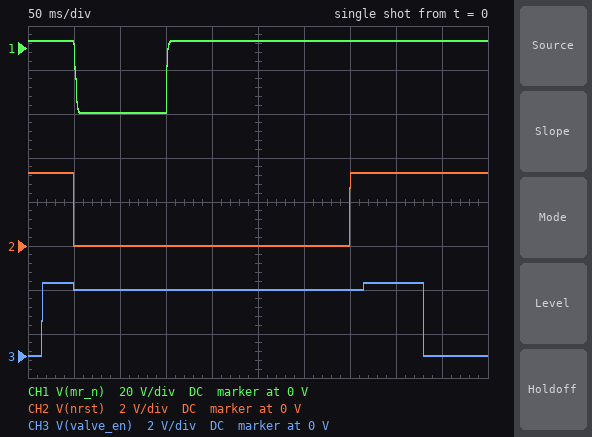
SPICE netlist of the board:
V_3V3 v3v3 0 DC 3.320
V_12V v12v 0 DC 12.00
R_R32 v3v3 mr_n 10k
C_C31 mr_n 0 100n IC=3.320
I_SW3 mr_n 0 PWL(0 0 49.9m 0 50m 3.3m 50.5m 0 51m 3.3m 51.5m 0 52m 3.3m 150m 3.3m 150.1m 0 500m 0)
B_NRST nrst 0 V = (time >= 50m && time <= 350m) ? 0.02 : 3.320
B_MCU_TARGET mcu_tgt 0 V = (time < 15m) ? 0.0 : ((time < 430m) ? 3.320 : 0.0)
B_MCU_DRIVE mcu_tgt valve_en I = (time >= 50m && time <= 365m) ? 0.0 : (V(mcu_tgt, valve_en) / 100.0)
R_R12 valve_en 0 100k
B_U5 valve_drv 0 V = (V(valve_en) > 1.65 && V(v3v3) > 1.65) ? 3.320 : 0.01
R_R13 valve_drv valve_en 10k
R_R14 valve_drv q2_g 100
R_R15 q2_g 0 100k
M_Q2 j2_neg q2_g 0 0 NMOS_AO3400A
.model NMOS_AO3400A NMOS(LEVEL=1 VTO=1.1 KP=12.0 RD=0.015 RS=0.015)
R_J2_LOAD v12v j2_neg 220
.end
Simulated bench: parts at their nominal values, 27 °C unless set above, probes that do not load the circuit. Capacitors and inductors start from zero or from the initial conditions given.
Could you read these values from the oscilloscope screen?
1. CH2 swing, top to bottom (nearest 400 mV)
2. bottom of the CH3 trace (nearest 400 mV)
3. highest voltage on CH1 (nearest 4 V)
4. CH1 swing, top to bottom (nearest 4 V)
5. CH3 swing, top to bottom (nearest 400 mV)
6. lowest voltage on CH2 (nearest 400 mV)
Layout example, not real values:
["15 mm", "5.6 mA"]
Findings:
["3.2 V", "0 V", "4 V", "32 V", "3.2 V", "0 V"]
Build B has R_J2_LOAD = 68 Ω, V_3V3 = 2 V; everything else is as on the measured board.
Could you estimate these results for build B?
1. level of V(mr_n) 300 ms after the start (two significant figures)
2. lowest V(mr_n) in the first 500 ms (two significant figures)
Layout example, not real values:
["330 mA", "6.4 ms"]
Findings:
["2.0 V", "-31 V"]
